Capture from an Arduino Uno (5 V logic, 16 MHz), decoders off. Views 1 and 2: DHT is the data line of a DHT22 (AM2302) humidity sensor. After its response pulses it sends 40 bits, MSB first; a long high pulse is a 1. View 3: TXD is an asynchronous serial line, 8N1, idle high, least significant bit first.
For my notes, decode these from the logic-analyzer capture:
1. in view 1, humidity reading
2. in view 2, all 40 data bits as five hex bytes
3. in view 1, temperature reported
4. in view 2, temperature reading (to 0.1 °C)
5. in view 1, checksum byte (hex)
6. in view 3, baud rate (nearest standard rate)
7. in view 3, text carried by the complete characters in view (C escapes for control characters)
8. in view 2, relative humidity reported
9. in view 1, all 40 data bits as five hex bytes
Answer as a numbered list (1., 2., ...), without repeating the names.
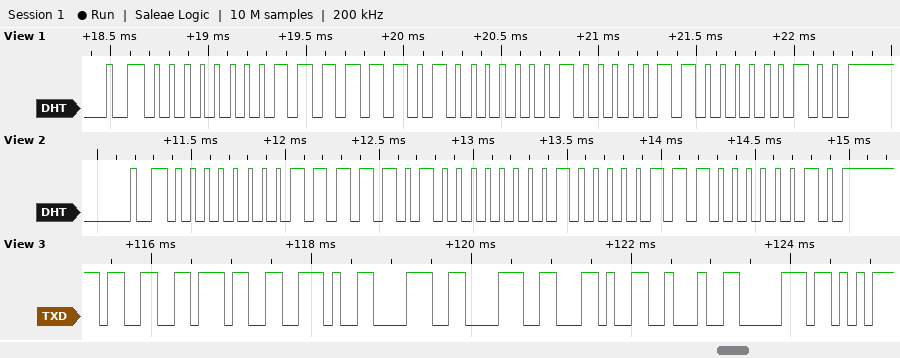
1. 25.3 %
2. 00 FA 01 07 02
3. 26.2 °C
4. 26.3 °C
5. 0x04
6. 9600 baud
7. "37.88,\"p"
8. 25.0 %
9. 00 FD 01 06 04
